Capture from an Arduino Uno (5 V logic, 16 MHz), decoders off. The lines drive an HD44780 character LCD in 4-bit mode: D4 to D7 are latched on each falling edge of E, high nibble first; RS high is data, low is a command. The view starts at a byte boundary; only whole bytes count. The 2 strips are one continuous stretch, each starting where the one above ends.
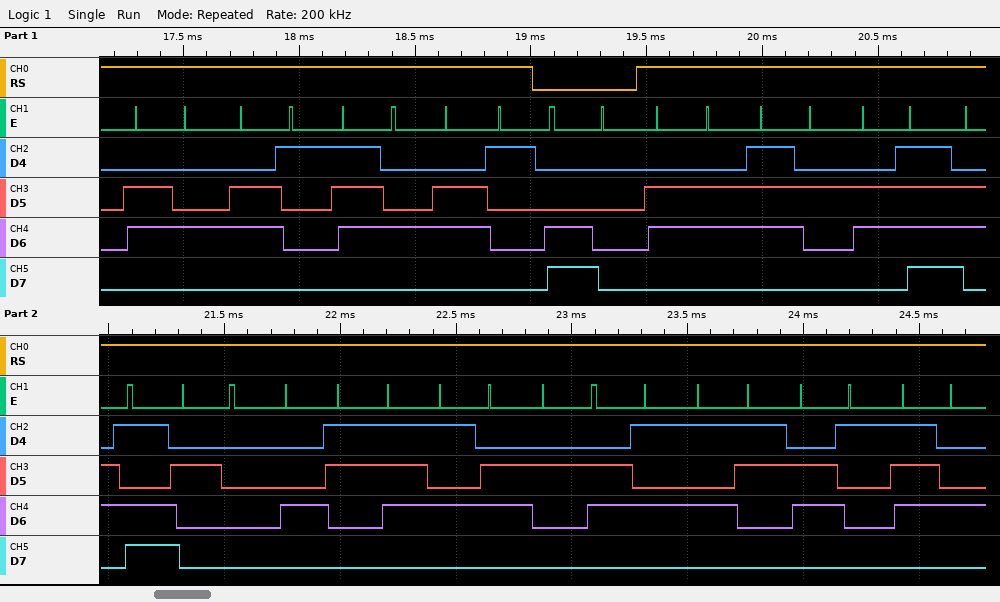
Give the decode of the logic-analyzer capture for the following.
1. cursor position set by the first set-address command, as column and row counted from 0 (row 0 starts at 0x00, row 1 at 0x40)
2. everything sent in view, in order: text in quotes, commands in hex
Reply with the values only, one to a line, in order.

column 0, row 1
"data" 0xC0 "from CubeSat"
